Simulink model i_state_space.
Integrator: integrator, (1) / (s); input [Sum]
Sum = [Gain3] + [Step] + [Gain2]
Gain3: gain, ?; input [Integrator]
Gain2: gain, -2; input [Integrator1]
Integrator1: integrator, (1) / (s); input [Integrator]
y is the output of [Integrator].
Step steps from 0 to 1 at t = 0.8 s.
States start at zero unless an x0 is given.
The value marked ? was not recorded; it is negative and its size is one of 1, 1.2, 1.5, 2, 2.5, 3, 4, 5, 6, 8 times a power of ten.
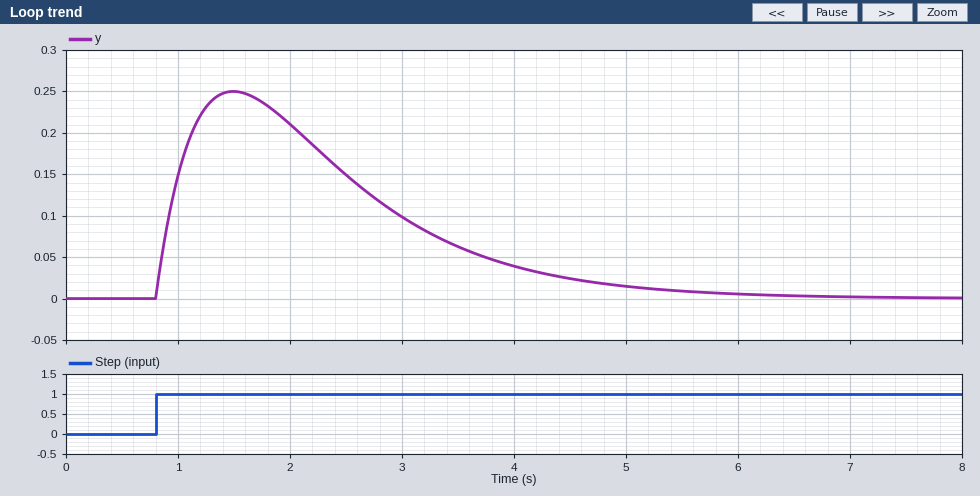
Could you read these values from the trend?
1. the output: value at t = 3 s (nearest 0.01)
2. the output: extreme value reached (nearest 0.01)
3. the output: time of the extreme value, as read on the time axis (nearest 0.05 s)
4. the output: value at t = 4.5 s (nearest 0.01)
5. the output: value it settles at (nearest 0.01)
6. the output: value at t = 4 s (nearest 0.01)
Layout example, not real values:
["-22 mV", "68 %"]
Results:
["0.10", "0.25", "1.50 s", "0.02", "0.00", "0.04"]
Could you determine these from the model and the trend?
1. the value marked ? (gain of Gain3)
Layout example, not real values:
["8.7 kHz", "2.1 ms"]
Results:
["-3"]
